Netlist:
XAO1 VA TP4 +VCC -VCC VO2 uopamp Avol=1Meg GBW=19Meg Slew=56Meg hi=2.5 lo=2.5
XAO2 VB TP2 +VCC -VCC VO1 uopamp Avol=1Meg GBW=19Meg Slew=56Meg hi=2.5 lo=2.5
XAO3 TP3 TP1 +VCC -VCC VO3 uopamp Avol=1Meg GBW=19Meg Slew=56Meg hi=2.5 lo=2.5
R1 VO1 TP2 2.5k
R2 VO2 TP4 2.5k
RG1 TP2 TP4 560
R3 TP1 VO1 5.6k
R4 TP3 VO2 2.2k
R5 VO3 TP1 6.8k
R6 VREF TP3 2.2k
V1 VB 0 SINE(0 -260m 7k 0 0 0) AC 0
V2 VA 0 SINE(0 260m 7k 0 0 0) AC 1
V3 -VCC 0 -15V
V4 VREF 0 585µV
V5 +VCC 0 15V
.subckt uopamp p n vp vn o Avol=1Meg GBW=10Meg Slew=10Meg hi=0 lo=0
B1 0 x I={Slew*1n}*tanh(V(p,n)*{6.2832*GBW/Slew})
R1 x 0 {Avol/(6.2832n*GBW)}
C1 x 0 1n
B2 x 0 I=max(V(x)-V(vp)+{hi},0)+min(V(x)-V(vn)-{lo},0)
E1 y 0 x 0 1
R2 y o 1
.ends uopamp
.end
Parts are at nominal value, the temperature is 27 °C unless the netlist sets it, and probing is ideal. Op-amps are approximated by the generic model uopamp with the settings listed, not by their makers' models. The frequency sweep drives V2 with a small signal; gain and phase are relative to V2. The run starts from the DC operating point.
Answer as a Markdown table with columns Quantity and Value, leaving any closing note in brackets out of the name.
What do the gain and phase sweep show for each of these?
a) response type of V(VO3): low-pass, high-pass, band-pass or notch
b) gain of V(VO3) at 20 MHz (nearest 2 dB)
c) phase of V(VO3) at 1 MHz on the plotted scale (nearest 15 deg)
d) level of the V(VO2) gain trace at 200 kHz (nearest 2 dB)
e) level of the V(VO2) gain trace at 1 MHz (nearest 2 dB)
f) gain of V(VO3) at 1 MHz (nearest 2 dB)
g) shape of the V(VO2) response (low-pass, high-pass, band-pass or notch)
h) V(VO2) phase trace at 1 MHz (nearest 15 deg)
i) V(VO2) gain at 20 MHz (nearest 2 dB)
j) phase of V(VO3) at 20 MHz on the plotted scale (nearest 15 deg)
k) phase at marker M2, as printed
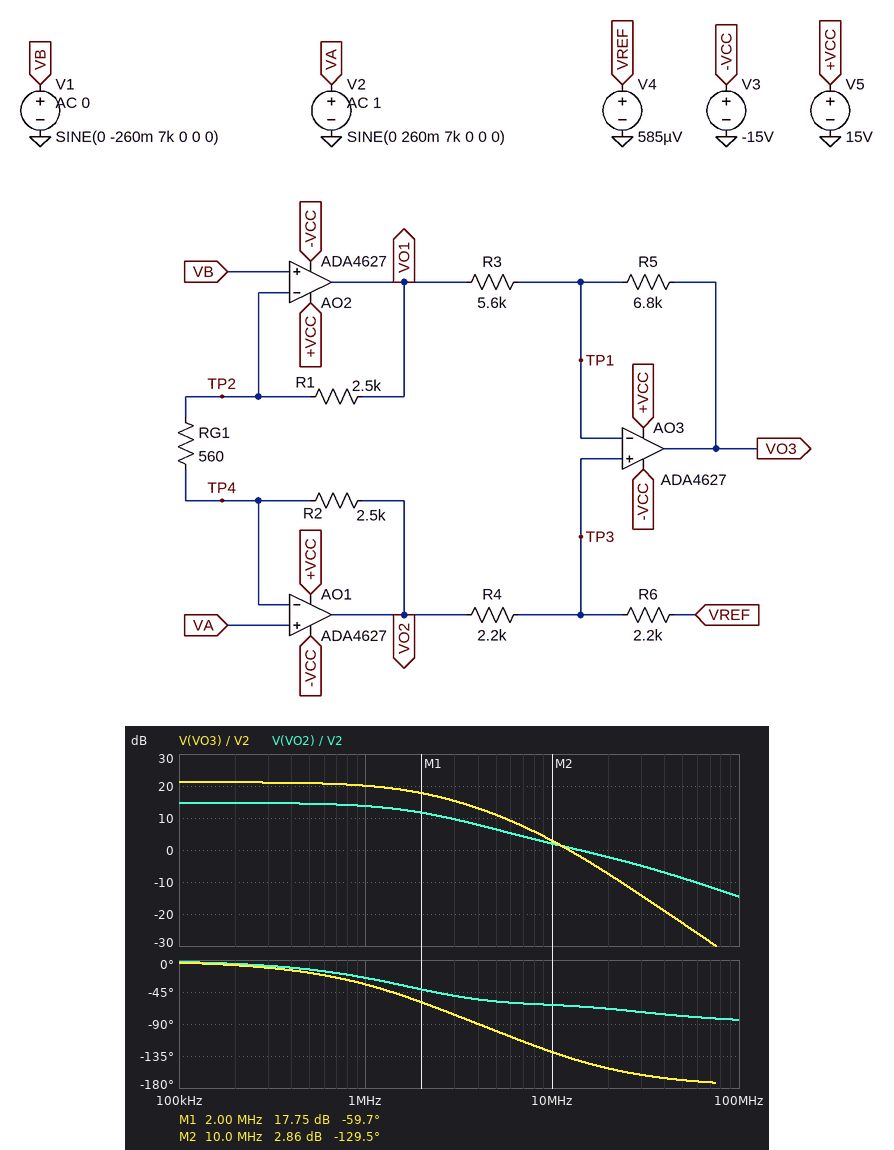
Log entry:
| Quantity | Value |
|---|---|
| response type of V(VO3): low-pass, high-pass, band-pass or notch | low-pass |
| gain of V(VO3) at 20 MHz | -8 dB |
| phase of V(VO3) at 1 MHz on the plotted scale | -30 deg |
| level of the V(VO2) gain trace at 200 kHz | 14 dB |
| level of the V(VO2) gain trace at 1 MHz | 14 dB |
| gain of V(VO3) at 1 MHz | 20 dB |
| shape of the V(VO2) response | low-pass |
| V(VO2) phase trace at 1 MHz | -30 deg |
| V(VO2) gain at 20 MHz | -2 dB |
| phase of V(VO3) at 20 MHz on the plotted scale | -150 deg |
| phase at marker M2, as printed | -129.5 deg |
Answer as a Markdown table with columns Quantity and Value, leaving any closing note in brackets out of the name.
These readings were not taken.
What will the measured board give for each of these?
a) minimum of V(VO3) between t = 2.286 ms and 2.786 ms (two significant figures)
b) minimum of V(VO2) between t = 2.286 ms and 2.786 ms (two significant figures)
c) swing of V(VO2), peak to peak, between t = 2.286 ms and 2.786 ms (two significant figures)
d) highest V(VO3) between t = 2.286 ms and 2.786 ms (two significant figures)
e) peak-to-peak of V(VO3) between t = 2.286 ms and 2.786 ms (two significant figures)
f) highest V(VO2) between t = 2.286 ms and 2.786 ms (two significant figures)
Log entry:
| Quantity | Value |
|---|---|
| minimum of V(VO3) between t = 2.286 ms and 2.786 ms | -6.0 V |
| minimum of V(VO2) between t = 2.286 ms and 2.786 ms | -2.6 V |
| swing of V(VO2), peak to peak, between t = 2.286 ms and 2.786 ms | 5.2 V |
| highest V(VO3) between t = 2.286 ms and 2.786 ms | 6.0 V |
| peak-to-peak of V(VO3) between t = 2.286 ms and 2.786 ms | 12 V |
| highest V(VO2) between t = 2.286 ms and 2.786 ms | 2.6 V |
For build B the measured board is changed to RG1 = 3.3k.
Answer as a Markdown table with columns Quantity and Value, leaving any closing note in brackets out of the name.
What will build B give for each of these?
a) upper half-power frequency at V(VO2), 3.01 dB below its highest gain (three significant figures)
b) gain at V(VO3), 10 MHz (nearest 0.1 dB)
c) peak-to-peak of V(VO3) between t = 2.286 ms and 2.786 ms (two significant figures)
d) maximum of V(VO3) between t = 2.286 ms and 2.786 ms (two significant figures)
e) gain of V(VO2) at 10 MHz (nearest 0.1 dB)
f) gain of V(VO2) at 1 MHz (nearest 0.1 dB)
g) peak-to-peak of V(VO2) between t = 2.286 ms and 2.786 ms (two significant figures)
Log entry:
| Quantity | Value |
|---|---|
| upper half-power frequency at V(VO2), 3.01 dB below its highest gain | 8.85 MHz |
| gain at V(VO3), 10 MHz | 1.0 dB |
| peak-to-peak of V(VO3) between t = 2.286 ms and 2.786 ms | 3.0 V |
| maximum of V(VO3) between t = 2.286 ms and 2.786 ms | 1.5 V |
| gain of V(VO2) at 10 MHz | 1.4 dB |
| gain of V(VO2) at 1 MHz | 4.8 dB |
| peak-to-peak of V(VO2) between t = 2.286 ms and 2.786 ms | 1.3 V |
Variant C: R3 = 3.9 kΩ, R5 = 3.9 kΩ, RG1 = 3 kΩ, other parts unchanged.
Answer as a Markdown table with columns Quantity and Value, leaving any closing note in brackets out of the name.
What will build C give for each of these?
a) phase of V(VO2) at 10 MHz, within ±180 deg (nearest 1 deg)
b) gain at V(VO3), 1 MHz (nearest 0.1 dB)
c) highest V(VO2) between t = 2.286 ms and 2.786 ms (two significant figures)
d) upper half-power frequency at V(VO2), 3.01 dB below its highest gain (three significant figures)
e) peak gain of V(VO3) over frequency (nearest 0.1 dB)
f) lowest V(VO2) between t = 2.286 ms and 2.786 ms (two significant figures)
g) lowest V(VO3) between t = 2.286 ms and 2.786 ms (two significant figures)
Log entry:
| Quantity | Value |
|---|---|
| phase of V(VO2) at 10 MHz, within ±180 deg | -45 deg |
| gain at V(VO3), 1 MHz | 8.4 dB |
| highest V(VO2) between t = 2.286 ms and 2.786 ms | 690 mV |
| upper half-power frequency at V(VO2), 3.01 dB below its highest gain | 8.30 MHz |
| peak gain of V(VO3) over frequency | 8.5 dB |
| lowest V(VO2) between t = 2.286 ms and 2.786 ms | -690 mV |
| lowest V(VO3) between t = 2.286 ms and 2.786 ms | -1.4 V |
